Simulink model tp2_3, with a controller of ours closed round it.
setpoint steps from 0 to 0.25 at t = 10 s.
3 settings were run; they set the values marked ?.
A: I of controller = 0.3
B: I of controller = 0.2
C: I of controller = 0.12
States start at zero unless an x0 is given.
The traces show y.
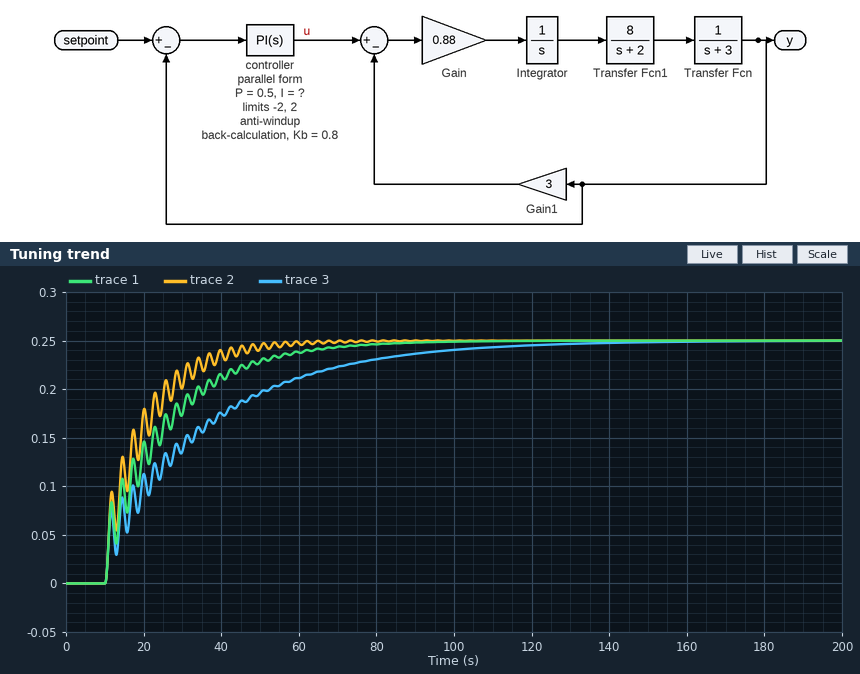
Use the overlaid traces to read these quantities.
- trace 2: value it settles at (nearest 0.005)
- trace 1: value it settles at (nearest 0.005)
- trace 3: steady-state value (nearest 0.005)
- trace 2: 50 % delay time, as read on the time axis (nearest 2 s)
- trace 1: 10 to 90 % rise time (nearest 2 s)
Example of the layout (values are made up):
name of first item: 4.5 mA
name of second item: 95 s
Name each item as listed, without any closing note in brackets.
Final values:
trace 2: value it settles at: 0.250
trace 1: value it settles at: 0.250
trace 3: steady-state value: 0.250
trace 2: 50 % delay time, as read on the time axis: 14 s
trace 1: 10 to 90 % rise time: 36 s
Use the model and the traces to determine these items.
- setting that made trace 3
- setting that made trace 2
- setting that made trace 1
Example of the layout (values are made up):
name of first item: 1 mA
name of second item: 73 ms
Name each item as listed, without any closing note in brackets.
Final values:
setting that made trace 3: C
setting that made trace 2: A
setting that made trace 1: B
